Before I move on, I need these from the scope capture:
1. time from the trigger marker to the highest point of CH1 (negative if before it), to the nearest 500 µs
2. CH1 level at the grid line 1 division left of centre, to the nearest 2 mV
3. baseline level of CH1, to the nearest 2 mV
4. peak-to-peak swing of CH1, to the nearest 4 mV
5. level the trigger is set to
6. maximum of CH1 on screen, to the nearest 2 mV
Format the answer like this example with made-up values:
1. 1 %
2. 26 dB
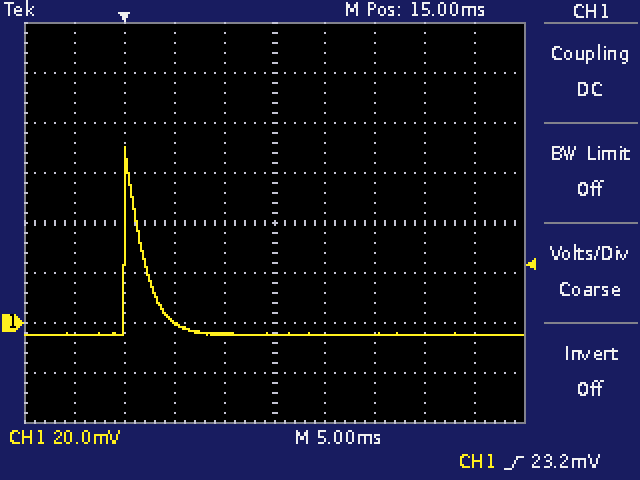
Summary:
1. 0.0 ms
2. -4 mV
3. -4 mV
4. 76 mV
5. 23.2 mV
6. 70 mV
